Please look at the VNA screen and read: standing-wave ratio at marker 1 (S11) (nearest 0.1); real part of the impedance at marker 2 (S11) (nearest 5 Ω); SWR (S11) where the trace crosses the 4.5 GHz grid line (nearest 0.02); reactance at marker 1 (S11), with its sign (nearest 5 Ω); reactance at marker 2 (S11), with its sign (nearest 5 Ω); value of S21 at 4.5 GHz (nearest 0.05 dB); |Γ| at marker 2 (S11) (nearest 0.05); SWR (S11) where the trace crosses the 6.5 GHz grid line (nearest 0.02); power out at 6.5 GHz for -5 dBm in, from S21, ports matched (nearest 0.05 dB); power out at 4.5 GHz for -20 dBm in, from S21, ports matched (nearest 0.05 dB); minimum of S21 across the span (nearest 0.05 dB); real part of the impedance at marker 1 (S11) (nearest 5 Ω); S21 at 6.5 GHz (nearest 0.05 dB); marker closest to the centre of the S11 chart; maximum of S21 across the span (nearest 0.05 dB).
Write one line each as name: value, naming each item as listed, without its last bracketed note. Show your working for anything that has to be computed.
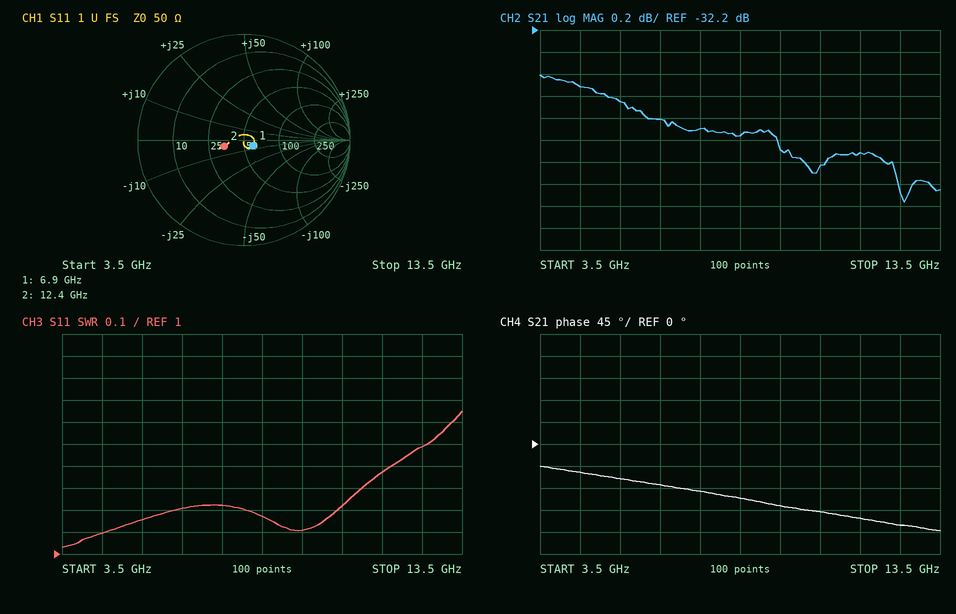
standing-wave ratio at marker 1 (S11): 1.2
real part of the impedance at marker 2 (S11): 35 Ω
SWR (S11) where the trace crosses the 4.5 GHz grid line: 1.10
reactance at marker 1 (S11), with its sign: -5 Ω
reactance at marker 2 (S11), with its sign: -5 Ω
value of S21 at 4.5 GHz: -32.70 dB
|Γ| at marker 2 (S11): 0.20
SWR (S11) where the trace crosses the 6.5 GHz grid line: 1.20
power out at 6.5 GHz for -5 dBm in, from S21, ports matched: -5 dBm + (-33.00 dB) = -38.00 dBm
power out at 4.5 GHz for -20 dBm in, from S21, ports matched: -20 dBm + (-32.70 dB) = -52.70 dBm
minimum of S21 across the span: -33.75 dB
real part of the impedance at marker 1 (S11): 60 Ω
S21 at 6.5 GHz: -33.00 dB
marker closest to the centre of the S11 chart: marker 1
maximum of S21 across the span: -32.60 dB
